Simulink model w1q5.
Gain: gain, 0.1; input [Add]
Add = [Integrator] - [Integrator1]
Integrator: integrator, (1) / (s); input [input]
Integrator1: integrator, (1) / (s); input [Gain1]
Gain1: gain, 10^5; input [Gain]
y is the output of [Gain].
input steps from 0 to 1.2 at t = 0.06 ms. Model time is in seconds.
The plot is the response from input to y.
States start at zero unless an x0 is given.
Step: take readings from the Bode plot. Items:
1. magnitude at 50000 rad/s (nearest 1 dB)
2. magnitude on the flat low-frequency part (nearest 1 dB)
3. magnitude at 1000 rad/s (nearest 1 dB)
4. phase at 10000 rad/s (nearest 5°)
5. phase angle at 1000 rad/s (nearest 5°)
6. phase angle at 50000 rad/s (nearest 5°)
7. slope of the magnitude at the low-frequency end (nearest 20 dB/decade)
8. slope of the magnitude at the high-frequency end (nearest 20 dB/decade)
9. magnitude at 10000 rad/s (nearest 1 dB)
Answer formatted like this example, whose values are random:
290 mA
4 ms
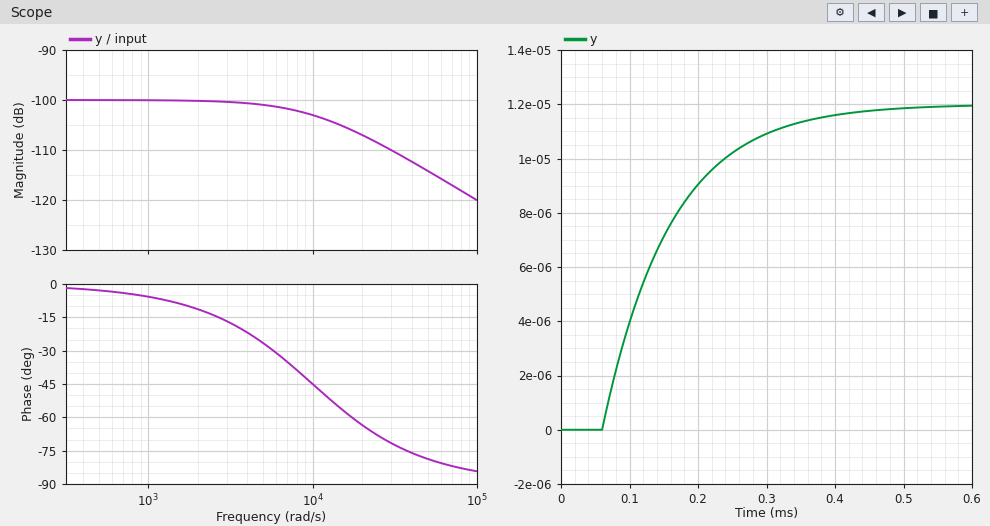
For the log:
-114 dB
-100 dB
-100 dB
-45°
-5°
-80°
0 dB/decade
-20 dB/decade
-103 dB
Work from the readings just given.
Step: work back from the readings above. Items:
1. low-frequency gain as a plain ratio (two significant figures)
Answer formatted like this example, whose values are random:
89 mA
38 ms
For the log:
0.000010
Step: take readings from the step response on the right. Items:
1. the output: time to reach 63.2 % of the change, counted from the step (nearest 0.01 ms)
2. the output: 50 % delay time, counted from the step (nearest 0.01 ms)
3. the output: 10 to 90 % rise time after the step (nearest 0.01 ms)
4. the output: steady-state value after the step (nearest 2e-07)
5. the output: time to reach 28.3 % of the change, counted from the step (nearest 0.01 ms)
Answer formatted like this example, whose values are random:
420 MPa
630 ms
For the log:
0.10 ms
0.07 ms
0.22 ms
0.0000120
0.03 ms
